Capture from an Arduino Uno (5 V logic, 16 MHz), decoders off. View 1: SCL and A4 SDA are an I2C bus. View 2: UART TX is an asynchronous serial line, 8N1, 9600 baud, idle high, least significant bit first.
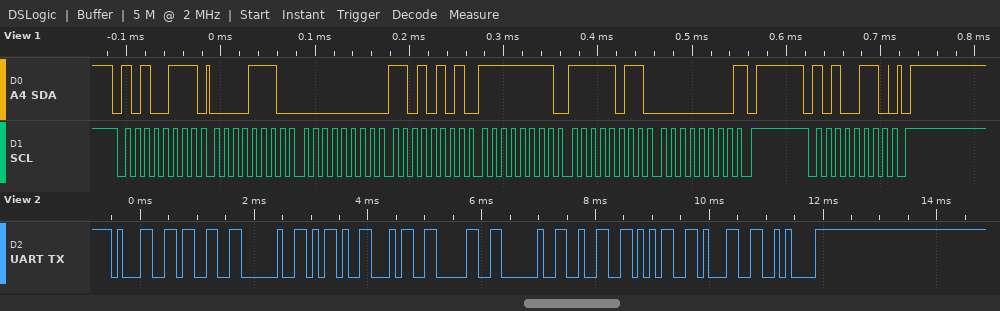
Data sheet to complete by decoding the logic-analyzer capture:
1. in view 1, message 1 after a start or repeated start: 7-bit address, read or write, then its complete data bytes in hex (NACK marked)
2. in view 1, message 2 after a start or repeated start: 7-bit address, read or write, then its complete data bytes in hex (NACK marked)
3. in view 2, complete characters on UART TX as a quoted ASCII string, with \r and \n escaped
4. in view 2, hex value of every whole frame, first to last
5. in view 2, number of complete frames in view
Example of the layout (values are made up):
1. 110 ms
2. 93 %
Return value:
1. 0x53 read: 0E 00 D5 FF FB 00 NACK
2. 0x53 write
3. "13 -40 251\n"
4. 0x31 0x33 0x20 0x2D 0x34 0x30 0x20 0x32 0x35 0x31 0x0A
5. 11
